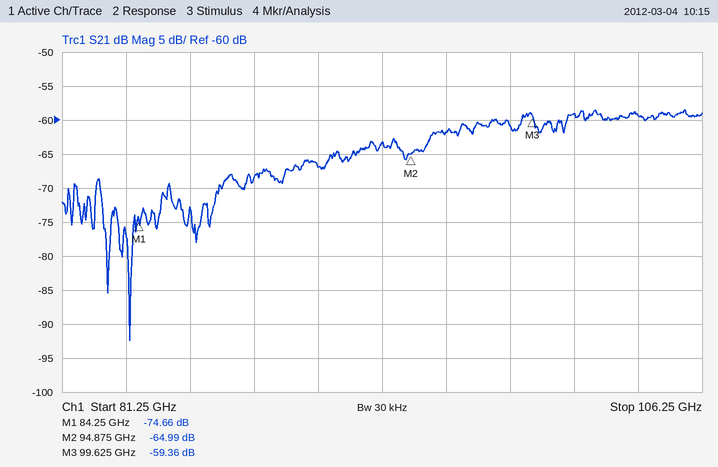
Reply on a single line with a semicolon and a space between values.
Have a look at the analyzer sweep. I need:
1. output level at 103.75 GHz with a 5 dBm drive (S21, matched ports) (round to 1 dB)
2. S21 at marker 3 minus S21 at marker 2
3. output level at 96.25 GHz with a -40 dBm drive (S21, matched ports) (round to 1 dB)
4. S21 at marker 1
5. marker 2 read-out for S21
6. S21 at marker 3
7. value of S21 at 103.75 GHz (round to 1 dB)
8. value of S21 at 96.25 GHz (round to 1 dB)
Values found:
-54 dBm; 5.63 dB; -102 dBm; -74.66 dB; -64.99 dB; -59.36 dB; -59 dB; -62 dB
